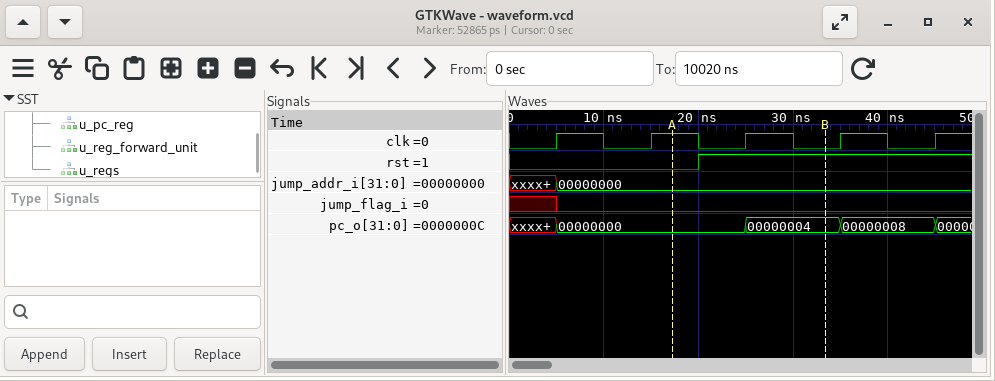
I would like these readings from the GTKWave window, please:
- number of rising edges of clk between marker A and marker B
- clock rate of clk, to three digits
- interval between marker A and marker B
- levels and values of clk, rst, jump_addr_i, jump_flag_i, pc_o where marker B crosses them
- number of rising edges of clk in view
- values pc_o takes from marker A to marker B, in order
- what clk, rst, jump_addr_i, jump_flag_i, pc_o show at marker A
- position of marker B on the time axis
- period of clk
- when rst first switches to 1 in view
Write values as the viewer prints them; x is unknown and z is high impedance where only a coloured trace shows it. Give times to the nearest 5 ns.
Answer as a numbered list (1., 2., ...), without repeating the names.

1. 1
2. 100 MHz
3. 15 ns
4. clk=0, rst=1, jump_addr_i=00000000, jump_flag_i=0, pc_o=00000004
5. 5
6. 00000000, 00000004
7. clk=1, rst=0, jump_addr_i=00000000, jump_flag_i=0, pc_o=00000000
8. 35 ns
9. 10 ns
10. 20 ns
